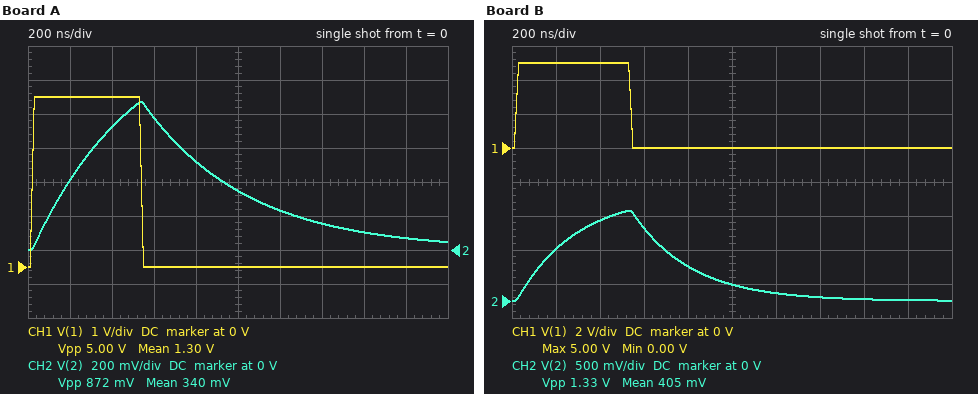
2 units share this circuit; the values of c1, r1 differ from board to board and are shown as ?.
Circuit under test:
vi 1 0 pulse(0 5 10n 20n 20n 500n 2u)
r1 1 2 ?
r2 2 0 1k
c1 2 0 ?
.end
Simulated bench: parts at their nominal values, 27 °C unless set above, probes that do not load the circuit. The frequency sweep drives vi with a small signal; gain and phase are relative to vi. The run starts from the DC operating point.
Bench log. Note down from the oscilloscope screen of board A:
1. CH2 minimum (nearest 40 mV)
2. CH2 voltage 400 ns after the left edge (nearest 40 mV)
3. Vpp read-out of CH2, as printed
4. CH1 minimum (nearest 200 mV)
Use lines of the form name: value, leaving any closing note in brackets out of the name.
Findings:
CH2 minimum: 0 V
CH2 voltage 400 ns after the left edge: 720 mV
Vpp read-out of CH2, as printed: 872 mV
CH1 minimum: 0 V
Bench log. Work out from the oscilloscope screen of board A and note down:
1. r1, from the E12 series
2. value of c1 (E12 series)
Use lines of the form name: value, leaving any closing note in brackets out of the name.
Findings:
r1, from the E12 series: 2.7 kΩ
value of c1: 680 pF
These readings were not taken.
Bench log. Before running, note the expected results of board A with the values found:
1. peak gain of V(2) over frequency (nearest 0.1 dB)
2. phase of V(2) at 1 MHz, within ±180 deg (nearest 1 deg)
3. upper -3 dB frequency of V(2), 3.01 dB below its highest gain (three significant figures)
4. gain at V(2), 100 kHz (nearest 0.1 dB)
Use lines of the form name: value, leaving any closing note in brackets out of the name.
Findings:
peak gain of V(2) over frequency: -11.4 dB
phase of V(2) at 1 MHz, within ±180 deg: -72 deg
upper -3 dB frequency of V(2), 3.01 dB below its highest gain: 321 kHz
gain at V(2), 100 kHz: -11.8 dB
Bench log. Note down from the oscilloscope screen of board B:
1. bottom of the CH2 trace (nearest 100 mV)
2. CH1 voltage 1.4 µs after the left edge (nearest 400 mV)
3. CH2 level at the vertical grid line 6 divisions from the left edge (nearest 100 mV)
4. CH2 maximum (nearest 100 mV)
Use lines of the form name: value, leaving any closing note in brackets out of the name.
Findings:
bottom of the CH2 trace: 0 V
CH1 voltage 1.4 µs after the left edge: 0 V
CH2 level at the vertical grid line 6 divisions from the left edge: 100 mV
CH2 maximum: 1.3 V
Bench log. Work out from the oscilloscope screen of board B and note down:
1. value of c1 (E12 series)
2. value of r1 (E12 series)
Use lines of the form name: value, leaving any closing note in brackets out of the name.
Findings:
value of c1: 390 pF
value of r1: 2.2 kΩ
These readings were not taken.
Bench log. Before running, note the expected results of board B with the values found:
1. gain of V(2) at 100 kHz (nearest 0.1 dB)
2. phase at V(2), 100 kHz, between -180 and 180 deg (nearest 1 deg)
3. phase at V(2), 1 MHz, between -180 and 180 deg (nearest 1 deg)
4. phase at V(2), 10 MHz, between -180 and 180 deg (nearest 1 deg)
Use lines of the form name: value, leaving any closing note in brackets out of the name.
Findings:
gain of V(2) at 100 kHz: -10.2 dB
phase at V(2), 100 kHz, between -180 and 180 deg: -10 deg
phase at V(2), 1 MHz, between -180 and 180 deg: -59 deg
phase at V(2), 10 MHz, between -180 and 180 deg: -87 deg
